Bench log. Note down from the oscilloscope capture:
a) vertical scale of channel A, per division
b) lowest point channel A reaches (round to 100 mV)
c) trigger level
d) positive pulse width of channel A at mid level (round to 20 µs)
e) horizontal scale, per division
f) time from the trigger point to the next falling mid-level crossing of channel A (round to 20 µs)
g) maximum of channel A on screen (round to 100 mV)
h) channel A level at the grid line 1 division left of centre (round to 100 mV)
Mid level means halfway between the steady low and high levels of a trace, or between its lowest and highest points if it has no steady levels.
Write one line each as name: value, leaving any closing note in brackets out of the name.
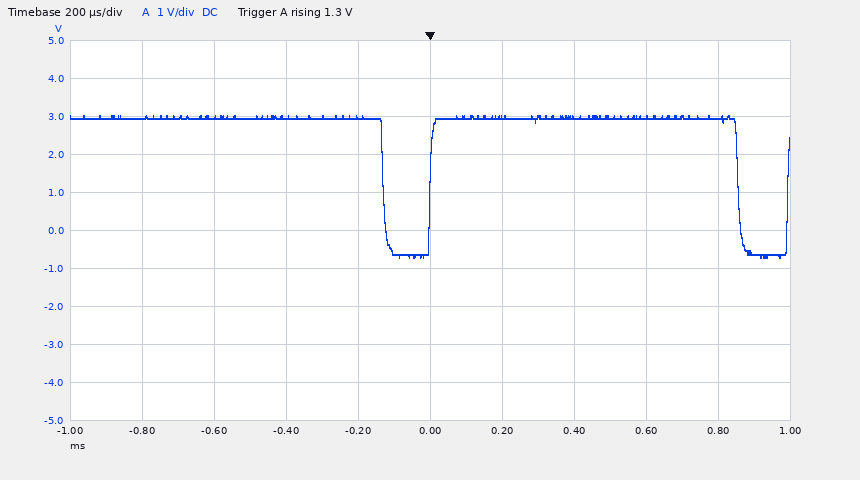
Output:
vertical scale of channel A, per division: 1 V
lowest point channel A reaches: -700 mV
trigger level: 1.3 V
positive pulse width of channel A at mid level: 860 µs
horizontal scale, per division: 200 µs
time from the trigger point to the next falling mid-level crossing of channel A: 860 µs
maximum of channel A on screen: 3.0 V
channel A level at the grid line 1 division left of centre: 3.0 V
